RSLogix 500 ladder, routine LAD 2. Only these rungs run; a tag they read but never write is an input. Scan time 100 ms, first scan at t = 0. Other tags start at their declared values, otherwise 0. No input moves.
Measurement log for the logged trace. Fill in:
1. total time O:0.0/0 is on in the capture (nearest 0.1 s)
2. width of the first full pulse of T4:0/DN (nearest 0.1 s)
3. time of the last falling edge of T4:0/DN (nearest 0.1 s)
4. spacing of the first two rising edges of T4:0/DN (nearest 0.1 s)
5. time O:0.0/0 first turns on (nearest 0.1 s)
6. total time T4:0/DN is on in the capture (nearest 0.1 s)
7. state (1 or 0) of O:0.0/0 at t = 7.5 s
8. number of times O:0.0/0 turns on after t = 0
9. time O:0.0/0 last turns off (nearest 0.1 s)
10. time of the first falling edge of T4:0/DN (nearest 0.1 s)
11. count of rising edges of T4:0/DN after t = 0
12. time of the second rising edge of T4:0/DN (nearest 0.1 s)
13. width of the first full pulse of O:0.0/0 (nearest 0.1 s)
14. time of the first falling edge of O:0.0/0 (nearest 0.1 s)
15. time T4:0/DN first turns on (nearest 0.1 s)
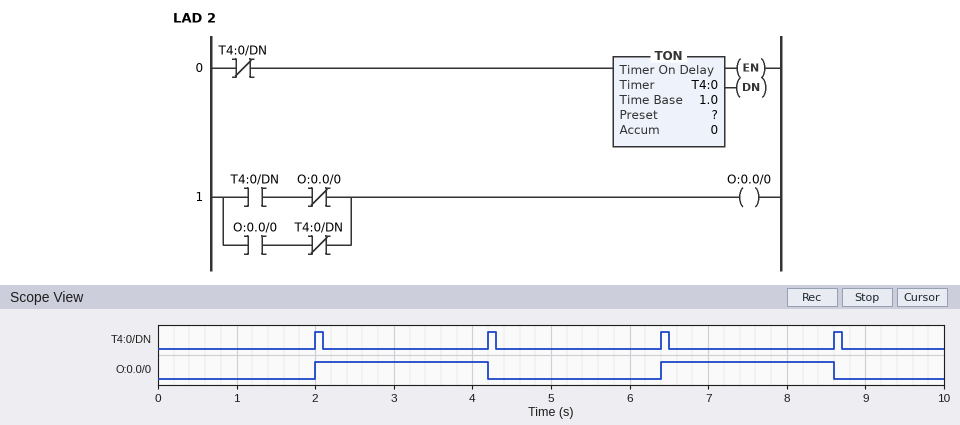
4.4 s
0.1 s
8.7 s
2.2 s
2.0 s
0.4 s
1
2
8.6 s
2.1 s
4
4.2 s
2.2 s
4.2 s
2.0 s
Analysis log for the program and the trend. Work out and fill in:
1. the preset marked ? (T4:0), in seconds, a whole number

2 s
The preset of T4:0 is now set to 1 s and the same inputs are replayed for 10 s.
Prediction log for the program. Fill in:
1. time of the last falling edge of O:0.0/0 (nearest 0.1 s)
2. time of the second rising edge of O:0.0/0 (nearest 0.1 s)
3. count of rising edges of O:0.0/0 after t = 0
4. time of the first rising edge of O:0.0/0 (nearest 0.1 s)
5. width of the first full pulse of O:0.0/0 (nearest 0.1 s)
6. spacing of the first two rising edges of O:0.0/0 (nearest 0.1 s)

9.4 s
3.4 s
4
1.0 s
1.2 s
2.4 s
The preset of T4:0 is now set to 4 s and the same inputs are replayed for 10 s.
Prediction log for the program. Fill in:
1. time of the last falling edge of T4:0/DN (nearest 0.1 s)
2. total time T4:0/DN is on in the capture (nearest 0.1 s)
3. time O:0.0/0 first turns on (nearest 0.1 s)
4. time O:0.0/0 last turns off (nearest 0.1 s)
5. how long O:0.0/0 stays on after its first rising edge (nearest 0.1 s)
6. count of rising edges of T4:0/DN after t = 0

8.3 s
0.2 s
4.0 s
8.2 s
4.2 s
2
